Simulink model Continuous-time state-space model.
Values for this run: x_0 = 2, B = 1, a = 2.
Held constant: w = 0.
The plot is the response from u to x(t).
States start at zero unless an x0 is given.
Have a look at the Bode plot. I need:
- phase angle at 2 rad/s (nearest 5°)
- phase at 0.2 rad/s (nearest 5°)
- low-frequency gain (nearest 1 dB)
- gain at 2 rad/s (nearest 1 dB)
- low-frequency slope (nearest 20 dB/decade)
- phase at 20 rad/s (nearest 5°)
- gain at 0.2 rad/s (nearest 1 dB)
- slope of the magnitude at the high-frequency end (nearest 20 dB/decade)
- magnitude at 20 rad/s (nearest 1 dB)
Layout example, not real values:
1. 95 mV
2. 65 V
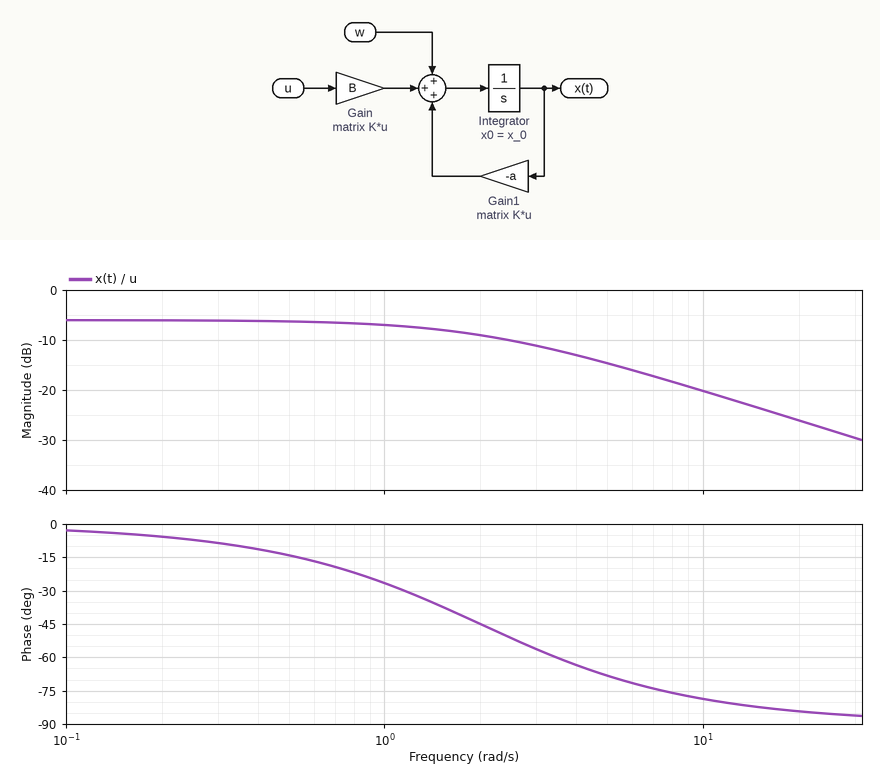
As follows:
1. -45°
2. -5°
3. -6 dB
4. -9 dB
5. 0 dB/decade
6. -85°
7. -6 dB
8. -20 dB/decade
9. -26 dB
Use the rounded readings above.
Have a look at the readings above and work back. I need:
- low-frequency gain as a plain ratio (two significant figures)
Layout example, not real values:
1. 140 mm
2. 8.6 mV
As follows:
1. 0.50
